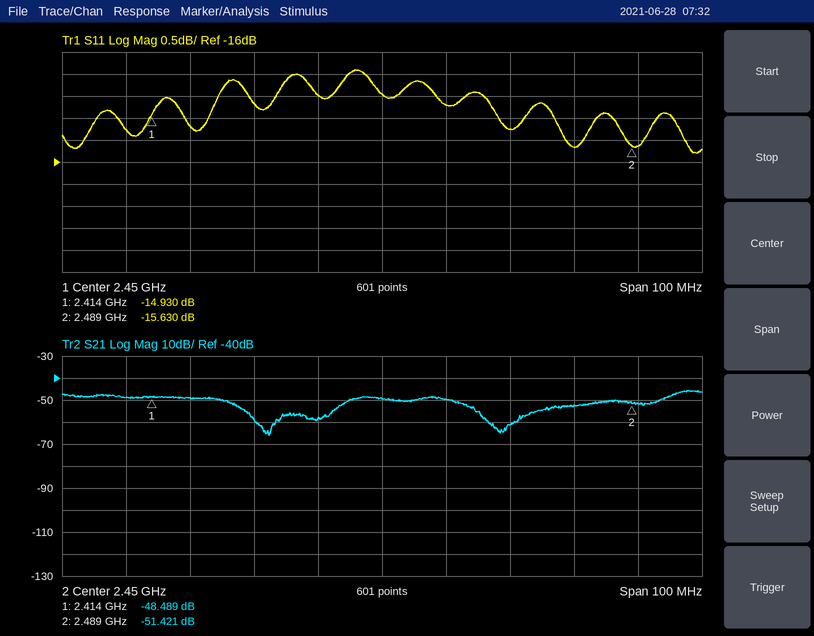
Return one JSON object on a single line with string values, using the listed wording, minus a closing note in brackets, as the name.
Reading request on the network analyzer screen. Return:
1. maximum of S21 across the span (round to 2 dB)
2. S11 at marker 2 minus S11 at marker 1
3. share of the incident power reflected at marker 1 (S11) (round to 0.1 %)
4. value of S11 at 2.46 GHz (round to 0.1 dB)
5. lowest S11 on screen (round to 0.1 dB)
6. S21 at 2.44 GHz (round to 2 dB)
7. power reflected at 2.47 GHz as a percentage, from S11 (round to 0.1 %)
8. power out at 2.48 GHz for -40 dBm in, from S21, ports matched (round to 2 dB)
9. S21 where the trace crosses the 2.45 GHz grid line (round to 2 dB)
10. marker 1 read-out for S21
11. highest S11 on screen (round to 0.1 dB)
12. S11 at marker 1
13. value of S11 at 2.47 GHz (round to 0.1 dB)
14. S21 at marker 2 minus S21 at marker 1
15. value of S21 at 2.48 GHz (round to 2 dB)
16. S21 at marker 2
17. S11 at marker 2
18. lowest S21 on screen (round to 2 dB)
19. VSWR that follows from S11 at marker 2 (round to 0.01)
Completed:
{"maximum of S21 across the span": "-46 dB", "S11 at marker 2 minus S11 at marker 1": "-0.700 dB", "share of the incident power reflected at marker 1 (S11)": "3.2 %", "value of S11 at 2.46 GHz": "-14.7 dB", "lowest S11 on screen": "-15.8 dB", "S21 at 2.44 GHz": "-58 dB", "power reflected at 2.47 GHz as a percentage, from S11": "3.0 %", "power out at 2.48 GHz for -40 dBm in, from S21, ports matched": "-92 dBm", "S21 where the trace crosses the 2.45 GHz grid line": "-50 dB", "marker 1 read-out for S21": "-48.489 dB", "highest S11 on screen": "-13.9 dB", "S11 at marker 1": "-14.930 dB", "value of S11 at 2.47 GHz": "-15.3 dB", "S21 at marker 2 minus S21 at marker 1": "-2.932 dB", "value of S21 at 2.48 GHz": "-52 dB", "S21 at marker 2": "-51.421 dB", "S11 at marker 2": "-15.630 dB", "lowest S21 on screen": "-66 dB", "VSWR that follows from S11 at marker 2": "1.40"}
